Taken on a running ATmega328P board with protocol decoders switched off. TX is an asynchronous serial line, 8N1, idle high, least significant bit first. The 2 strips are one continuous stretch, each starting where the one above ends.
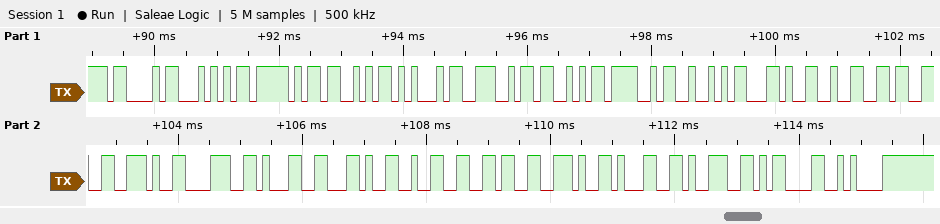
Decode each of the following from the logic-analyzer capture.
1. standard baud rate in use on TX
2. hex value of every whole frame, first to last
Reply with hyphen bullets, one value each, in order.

- 9600 baud
- 43 54 5F 53 45 4E 53 4F 52 2C 32 33 2E 38 31 2C 32 36 2E 31 39 0D 0A
